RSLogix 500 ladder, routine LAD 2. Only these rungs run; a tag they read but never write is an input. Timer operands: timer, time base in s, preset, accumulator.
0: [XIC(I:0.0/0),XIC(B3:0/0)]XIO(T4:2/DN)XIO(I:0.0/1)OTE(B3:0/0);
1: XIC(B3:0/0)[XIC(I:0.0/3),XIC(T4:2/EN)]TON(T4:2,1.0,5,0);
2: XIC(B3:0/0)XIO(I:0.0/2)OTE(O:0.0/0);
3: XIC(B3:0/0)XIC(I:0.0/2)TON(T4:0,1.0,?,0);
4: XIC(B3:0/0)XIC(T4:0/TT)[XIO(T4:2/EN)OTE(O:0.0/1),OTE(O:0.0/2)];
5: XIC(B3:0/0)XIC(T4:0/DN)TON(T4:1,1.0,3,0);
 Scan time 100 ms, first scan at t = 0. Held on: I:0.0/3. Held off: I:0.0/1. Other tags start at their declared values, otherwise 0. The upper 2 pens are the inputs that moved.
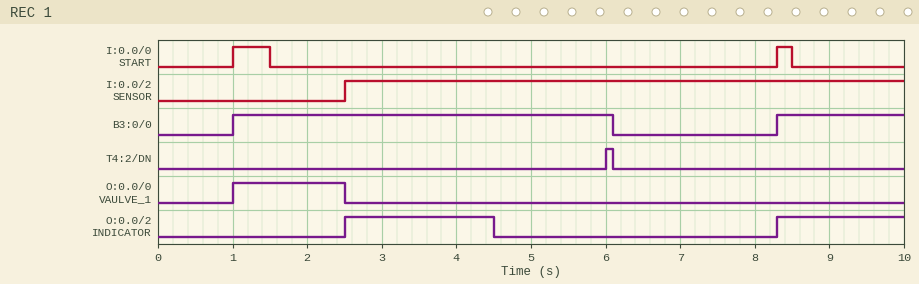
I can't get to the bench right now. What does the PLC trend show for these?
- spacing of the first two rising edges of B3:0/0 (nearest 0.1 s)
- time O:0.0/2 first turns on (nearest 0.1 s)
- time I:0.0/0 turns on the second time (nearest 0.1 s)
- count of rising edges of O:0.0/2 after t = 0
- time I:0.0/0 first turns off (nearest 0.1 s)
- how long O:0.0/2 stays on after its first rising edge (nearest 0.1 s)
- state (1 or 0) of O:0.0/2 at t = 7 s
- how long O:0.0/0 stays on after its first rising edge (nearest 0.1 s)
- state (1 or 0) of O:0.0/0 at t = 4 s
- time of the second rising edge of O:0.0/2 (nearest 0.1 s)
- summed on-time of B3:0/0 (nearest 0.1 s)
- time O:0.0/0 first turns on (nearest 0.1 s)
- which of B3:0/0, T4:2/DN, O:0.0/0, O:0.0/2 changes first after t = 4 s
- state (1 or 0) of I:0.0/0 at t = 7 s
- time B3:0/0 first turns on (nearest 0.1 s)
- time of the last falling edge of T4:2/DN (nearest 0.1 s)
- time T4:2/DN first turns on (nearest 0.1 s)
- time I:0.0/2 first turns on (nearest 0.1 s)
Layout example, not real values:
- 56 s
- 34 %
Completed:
- 7.3 s
- 2.5 s
- 8.3 s
- 2
- 1.5 s
- 2.0 s
- 0
- 1.5 s
- 0
- 8.3 s
- 6.8 s
- 1.0 s
- O:0.0/2
- 0
- 1.0 s
- 6.1 s
- 6.0 s
- 2.5 s
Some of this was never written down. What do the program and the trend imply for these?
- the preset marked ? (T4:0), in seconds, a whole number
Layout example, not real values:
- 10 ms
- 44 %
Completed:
- 2 s
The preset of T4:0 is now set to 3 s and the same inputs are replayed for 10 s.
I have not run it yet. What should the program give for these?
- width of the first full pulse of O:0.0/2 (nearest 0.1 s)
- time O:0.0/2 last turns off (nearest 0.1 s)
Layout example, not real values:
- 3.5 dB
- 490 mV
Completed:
- 3.0 s
- 5.5 s
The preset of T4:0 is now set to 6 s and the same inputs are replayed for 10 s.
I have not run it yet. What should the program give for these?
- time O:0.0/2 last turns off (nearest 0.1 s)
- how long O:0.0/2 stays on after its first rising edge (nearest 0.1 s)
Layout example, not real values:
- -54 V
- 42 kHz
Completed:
- 6.1 s
- 3.6 s
